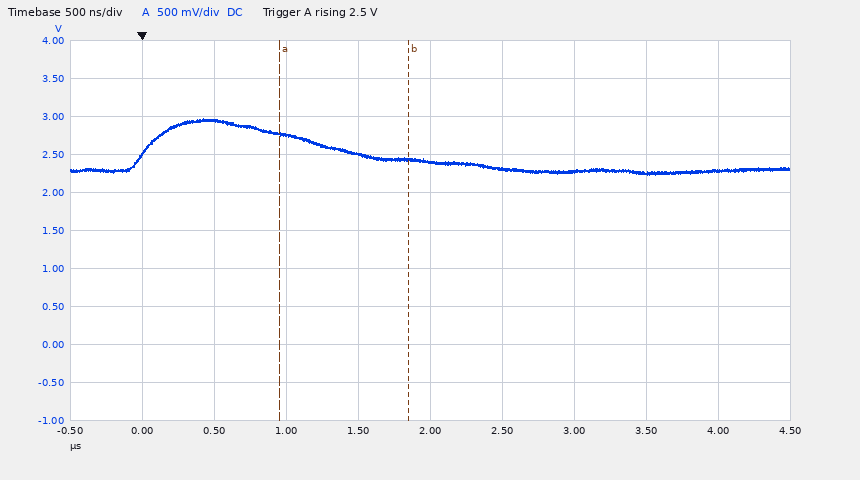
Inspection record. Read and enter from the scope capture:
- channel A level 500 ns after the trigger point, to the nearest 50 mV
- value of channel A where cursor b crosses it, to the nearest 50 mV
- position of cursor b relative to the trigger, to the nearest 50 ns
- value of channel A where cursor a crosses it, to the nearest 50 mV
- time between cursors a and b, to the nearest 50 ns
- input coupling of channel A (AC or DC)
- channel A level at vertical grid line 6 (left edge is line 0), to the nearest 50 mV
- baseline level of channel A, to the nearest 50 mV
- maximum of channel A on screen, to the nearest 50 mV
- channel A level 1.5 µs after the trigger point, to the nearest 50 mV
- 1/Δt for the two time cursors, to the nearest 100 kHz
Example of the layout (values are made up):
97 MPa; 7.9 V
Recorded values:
2.95 V; 2.45 V; +1.85 µs; 2.75 V; 900 ns; DC; 2.30 V; 2.30 V; 2.95 V; 2.50 V; 1.1 MHz
